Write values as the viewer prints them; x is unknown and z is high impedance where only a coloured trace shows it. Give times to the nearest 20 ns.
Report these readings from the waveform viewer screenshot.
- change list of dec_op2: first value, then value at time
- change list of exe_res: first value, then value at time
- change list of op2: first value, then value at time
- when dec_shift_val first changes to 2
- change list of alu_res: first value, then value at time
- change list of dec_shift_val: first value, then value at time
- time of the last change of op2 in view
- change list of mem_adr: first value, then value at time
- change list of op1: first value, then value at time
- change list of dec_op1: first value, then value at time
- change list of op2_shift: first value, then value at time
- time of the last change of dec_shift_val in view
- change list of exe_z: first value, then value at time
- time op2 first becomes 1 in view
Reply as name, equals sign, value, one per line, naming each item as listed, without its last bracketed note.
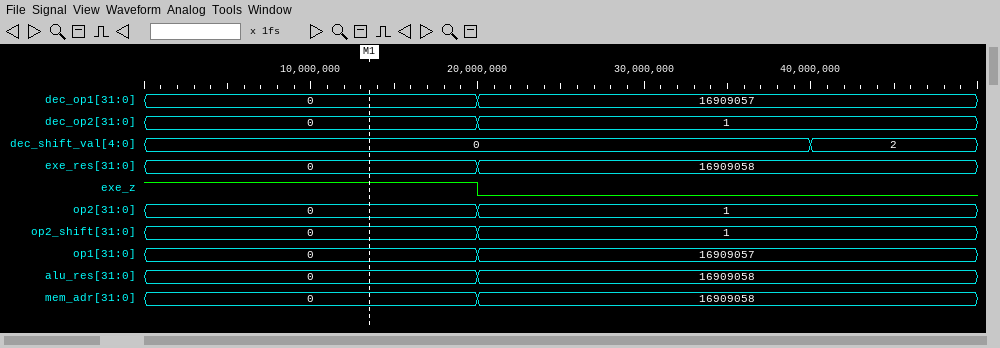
change list of dec_op2: first value, then value at time = 0, 1 at 20 ns
change list of exe_res: first value, then value at time = 0, 16909058 at 20 ns
change list of op2: first value, then value at time = 0, 1 at 20 ns
when dec_shift_val first changes to 2 = 40 ns
change list of alu_res: first value, then value at time = 0, 16909058 at 20 ns
change list of dec_shift_val: first value, then value at time = 0, 2 at 40 ns
time of the last change of op2 in view = 20 ns
change list of mem_adr: first value, then value at time = 0, 16909058 at 20 ns
change list of op1: first value, then value at time = 0, 16909057 at 20 ns
change list of dec_op1: first value, then value at time = 0, 16909057 at 20 ns
change list of op2_shift: first value, then value at time = 0, 1 at 20 ns
time of the last change of dec_shift_val in view = 40 ns
change list of exe_z: first value, then value at time = 1, 0 at 20 ns
time op2 first becomes 1 in view = 20 ns
